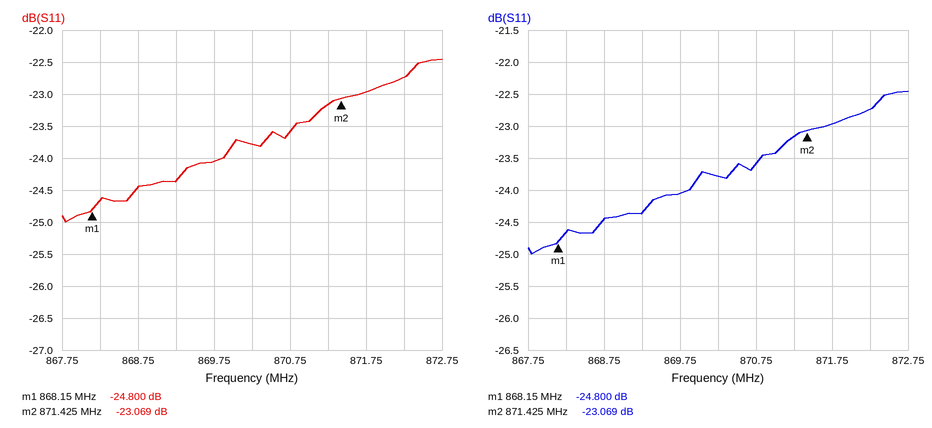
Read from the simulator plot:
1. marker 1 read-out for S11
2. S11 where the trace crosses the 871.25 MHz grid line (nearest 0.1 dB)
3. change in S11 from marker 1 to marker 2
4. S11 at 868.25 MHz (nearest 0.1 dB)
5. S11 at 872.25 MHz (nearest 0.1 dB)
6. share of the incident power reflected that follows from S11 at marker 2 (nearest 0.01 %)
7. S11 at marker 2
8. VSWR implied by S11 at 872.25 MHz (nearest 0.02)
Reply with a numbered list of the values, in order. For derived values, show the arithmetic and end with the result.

1. -24.800 dB
2. -23.2 dB
3. -23.069 − (-24.8) = 1.731 dB
4. -24.7 dB
5. -22.7 dB
6. 10^(-23.069/10) ≈ 0.49 %
7. -23.069 dB
8. |Γ| = 10^(-22.7/20) = 0.0733; VSWR = (1 + 0.0733)/(1 − 0.0733) ≈ 1.16
